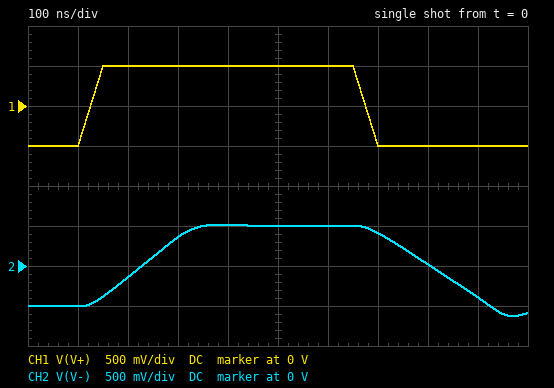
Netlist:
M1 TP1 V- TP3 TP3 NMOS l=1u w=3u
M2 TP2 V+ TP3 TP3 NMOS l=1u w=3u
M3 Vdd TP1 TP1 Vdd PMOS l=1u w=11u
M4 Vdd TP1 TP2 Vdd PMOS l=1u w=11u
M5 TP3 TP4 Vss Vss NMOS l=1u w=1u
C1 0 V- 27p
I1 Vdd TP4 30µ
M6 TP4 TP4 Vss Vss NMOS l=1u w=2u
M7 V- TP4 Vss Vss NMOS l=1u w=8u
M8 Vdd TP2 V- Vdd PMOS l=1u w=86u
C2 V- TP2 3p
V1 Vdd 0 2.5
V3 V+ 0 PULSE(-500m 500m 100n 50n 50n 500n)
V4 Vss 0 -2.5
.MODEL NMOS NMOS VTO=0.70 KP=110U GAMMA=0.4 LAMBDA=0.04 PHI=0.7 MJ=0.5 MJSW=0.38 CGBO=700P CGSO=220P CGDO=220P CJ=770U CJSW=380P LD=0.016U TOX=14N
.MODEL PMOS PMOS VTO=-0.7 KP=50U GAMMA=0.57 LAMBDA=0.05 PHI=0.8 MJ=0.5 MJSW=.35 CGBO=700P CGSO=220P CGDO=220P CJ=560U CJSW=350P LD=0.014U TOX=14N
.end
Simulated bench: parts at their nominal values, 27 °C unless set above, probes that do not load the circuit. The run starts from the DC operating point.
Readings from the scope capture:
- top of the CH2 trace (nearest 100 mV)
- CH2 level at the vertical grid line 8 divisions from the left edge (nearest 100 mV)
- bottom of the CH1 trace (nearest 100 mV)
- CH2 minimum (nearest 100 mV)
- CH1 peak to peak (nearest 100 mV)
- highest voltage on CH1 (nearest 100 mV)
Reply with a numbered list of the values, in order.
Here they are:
1. 500 mV
2. 0 V
3. -500 mV
4. -600 mV
5. 1.0 V
6. 500 mV
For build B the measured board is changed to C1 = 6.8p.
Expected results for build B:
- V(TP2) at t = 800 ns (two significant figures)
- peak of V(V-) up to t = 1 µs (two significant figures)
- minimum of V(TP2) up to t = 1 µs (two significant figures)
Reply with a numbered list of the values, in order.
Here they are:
1. 1.6 V
2. 500 mV
3. 1.5 V
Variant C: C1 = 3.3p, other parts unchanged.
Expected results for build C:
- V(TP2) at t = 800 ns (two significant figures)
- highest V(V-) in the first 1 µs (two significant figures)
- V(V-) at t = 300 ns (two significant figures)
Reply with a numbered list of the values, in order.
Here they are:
1. 1.6 V
2. 500 mV
3. 410 mV
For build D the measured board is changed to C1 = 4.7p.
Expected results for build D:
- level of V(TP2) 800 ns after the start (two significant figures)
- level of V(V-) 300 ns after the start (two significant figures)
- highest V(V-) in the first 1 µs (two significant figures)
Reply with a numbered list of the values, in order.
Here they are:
1. 1.6 V
2. 410 mV
3. 500 mV
